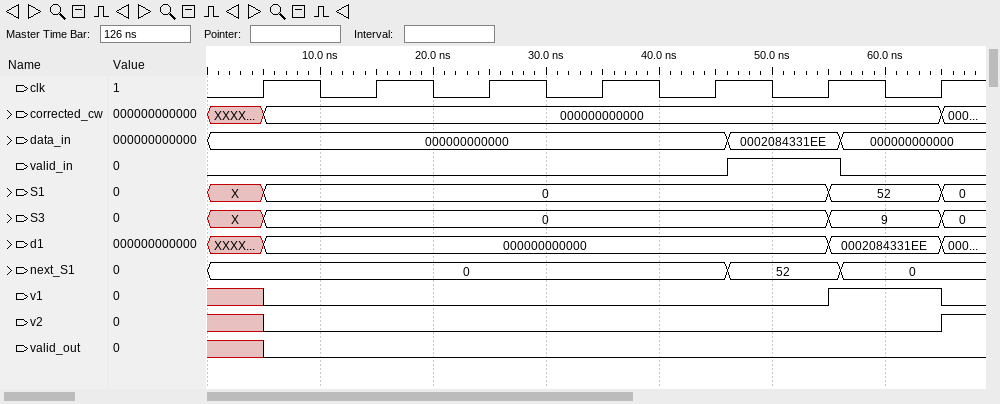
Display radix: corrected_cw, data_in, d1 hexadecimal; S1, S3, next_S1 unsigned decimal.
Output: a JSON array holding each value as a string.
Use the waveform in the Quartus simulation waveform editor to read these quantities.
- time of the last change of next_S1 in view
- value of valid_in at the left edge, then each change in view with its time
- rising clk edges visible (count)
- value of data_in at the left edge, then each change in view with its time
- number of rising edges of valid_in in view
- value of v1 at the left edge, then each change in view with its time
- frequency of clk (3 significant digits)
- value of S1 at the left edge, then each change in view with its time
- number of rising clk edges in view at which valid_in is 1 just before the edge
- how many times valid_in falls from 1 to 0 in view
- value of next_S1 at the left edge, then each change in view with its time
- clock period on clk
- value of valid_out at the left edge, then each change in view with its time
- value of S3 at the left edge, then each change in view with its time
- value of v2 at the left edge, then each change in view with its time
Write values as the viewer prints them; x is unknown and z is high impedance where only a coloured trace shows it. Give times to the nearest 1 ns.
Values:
["56 ns", "0, 1 at 46 ns, 0 at 56 ns", "7", "000000000000, 0002084331EE at 46 ns, 000000000000 at 56 ns", "1", "x, 0 at 5 ns, 1 at 55 ns, 0 at 65 ns", "100 MHz", "X, 0 at 5 ns, 52 at 55 ns, 0 at 65 ns", "1", "1", "0, 52 at 46 ns, 0 at 56 ns", "10 ns", "x, 0 at 5 ns", "X, 0 at 5 ns, 9 at 55 ns, 0 at 65 ns", "x, 0 at 5 ns, 1 at 65 ns"]
